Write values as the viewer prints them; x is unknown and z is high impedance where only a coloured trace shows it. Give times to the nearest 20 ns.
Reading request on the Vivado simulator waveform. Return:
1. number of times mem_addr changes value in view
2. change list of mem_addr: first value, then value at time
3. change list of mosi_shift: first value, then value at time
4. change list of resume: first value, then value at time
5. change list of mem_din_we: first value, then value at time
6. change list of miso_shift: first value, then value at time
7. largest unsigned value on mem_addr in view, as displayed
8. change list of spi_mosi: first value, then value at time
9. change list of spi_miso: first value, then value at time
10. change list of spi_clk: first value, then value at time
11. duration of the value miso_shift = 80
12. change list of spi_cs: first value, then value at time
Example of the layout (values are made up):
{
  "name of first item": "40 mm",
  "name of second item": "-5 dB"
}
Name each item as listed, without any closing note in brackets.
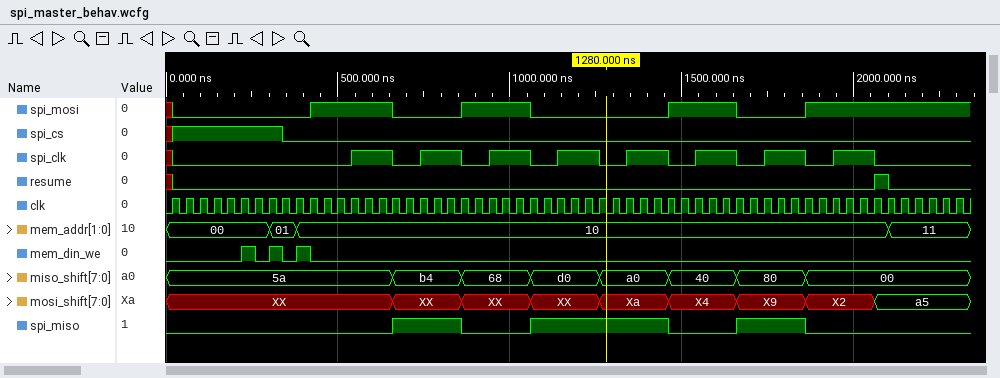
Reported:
{
  "number of times mem_addr changes value in view": "3",
  "change list of mem_addr: first value, then value at time": "00, 01 at 300 ns, 10 at 380 ns, 11 at 2100 ns",
  "change list of mosi_shift: first value, then value at time": "XX, XX at 660 ns, XX at 860 ns, XX at 1060 ns, Xa at 1260 ns, X4 at 1460 ns, X9 at 1660 ns, X2 at 1860 ns, a5 at 2060 ns",
  "change list of resume: first value, then value at time": "x, 0 at 20 ns, 1 at 2060 ns, 0 at 2100 ns",
  "change list of mem_din_we: first value, then value at time": "0, 1 at 220 ns, 0 at 260 ns, 1 at 300 ns, 0 at 340 ns, 1 at 380 ns, 0 at 420 ns",
  "change list of miso_shift: first value, then value at time": "5a, b4 at 660 ns, 68 at 860 ns, d0 at 1060 ns, a0 at 1260 ns, 40 at 1460 ns, 80 at 1660 ns, 00 at 1860 ns",
  "largest unsigned value on mem_addr in view, as displayed": "11",
  "change list of spi_mosi: first value, then value at time": "x, 0 at 20 ns, 1 at 420 ns, 0 at 660 ns, 1 at 860 ns, 0 at 1060 ns, 1 at 1460 ns, 0 at 1660 ns, 1 at 1860 ns",
  "change list of spi_miso: first value, then value at time": "0, 1 at 660 ns, 0 at 860 ns, 1 at 1060 ns, 0 at 1460 ns, 1 at 1660 ns, 0 at 1860 ns",
  "change list of spi_clk: first value, then value at time": "x, 0 at 20 ns, 1 at 540 ns, 0 at 660 ns, 1 at 740 ns, 0 at 860 ns, 1 at 940 ns, 0 at 1060 ns, 1 at 1140 ns, 0 at 1260 ns, 1 at 1340 ns, 0 at 1460 ns, 1 at 1540 ns, 0 at 1660 ns, 1 at 1740 ns, 0 at 1860 ns, 1 at 1940 ns, 0 at 2060 ns",
  "duration of the value miso_shift = 80": "200 ns",
  "change list of spi_cs: first value, then value at time": "x, 1 at 20 ns, 0 at 340 ns"
}
